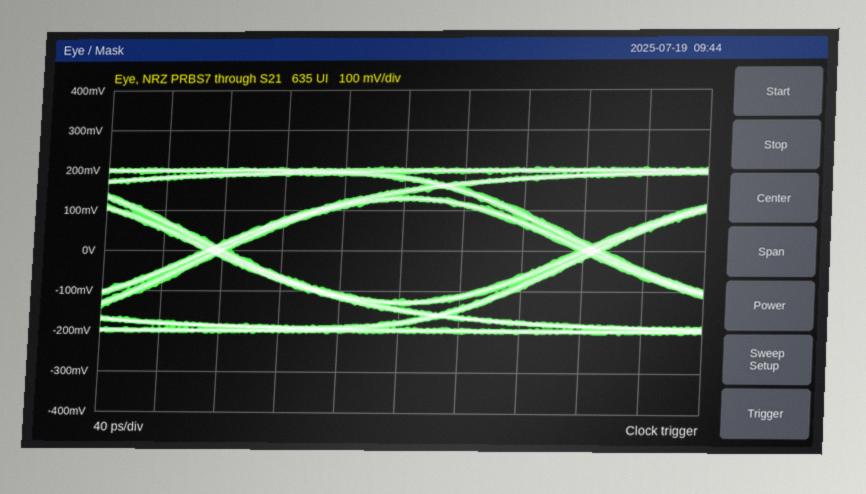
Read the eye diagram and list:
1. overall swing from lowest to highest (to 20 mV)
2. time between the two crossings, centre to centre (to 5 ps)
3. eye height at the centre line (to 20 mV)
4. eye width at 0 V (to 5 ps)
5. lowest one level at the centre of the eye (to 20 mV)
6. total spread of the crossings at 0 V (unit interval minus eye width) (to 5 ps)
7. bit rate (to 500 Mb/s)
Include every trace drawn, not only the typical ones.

420 mV
250 ps
240 mV
230 ps
120 mV
20 ps
4.0 Gb/s
